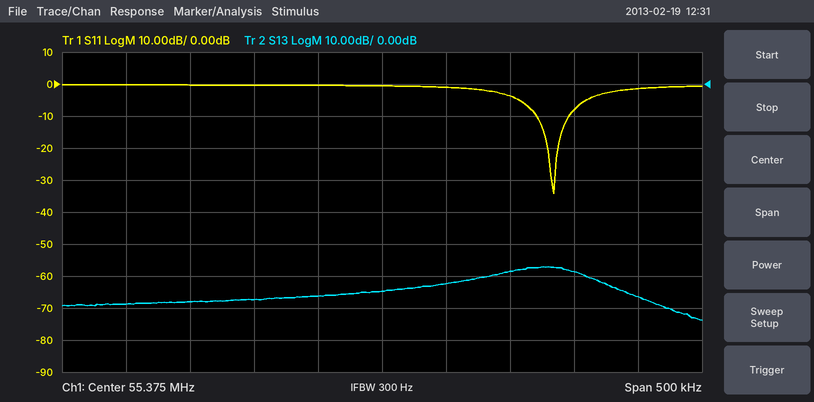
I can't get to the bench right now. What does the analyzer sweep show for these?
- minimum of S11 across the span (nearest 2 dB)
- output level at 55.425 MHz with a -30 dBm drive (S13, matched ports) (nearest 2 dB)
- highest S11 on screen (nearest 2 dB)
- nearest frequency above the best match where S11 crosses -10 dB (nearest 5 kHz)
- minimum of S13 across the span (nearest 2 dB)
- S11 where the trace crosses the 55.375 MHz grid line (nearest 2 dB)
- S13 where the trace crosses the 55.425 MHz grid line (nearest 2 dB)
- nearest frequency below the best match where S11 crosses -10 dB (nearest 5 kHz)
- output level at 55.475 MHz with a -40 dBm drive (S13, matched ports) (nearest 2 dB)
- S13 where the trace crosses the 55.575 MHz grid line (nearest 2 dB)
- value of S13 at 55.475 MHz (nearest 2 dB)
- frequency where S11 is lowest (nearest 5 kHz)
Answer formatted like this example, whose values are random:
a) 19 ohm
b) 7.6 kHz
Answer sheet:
a) -34 dB
b) -92 dBm
c) 0 dB
d) 55.520 MHz
e) -74 dB
f) 0 dB
g) -62 dB
h) 55.495 MHz
i) -98 dBm
j) -66 dB
k) -58 dB
l) 55.510 MHz
